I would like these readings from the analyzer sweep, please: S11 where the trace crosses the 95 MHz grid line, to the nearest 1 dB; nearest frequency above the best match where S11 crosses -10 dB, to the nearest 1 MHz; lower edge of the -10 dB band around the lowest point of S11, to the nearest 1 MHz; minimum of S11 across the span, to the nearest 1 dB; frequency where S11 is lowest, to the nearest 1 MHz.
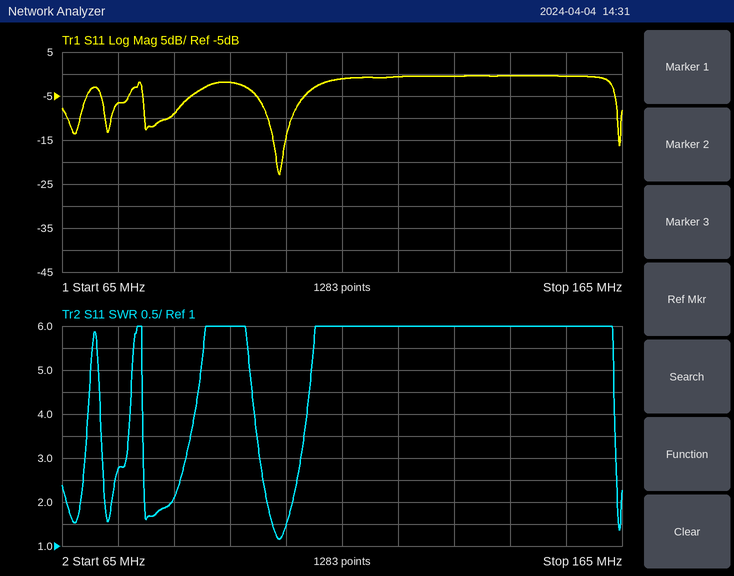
-2 dB
106 MHz
102 MHz
-23 dB
104 MHz
